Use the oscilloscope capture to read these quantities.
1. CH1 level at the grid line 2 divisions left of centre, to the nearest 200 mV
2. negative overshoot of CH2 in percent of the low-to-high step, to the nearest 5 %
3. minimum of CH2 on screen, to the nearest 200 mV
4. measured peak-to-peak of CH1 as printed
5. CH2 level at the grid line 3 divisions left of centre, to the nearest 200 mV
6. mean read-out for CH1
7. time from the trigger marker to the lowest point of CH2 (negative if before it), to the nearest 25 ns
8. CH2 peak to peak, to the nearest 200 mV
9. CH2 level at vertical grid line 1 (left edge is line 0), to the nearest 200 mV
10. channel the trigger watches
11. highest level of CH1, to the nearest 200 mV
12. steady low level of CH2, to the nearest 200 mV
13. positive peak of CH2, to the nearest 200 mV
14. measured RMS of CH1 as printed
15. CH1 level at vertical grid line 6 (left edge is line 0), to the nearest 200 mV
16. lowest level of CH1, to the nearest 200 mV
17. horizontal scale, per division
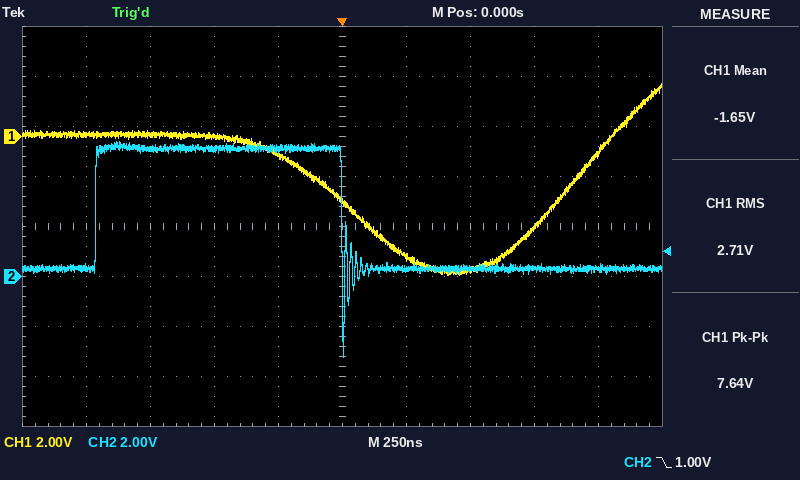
0.0 V
75 %
-3.2 V
7.64 V
5.2 V
-1.65 V
0 ns
8.6 V
400 mV
CH2
2.2 V
400 mV
5.4 V
2.71 V
-4.8 V
-5.6 V
250 ns
